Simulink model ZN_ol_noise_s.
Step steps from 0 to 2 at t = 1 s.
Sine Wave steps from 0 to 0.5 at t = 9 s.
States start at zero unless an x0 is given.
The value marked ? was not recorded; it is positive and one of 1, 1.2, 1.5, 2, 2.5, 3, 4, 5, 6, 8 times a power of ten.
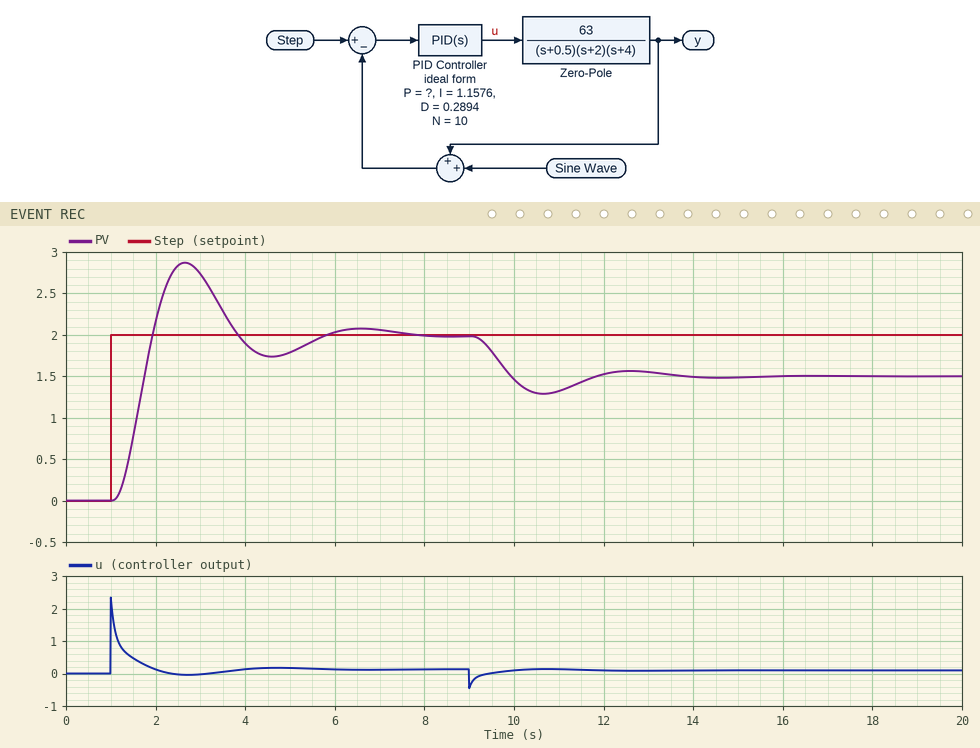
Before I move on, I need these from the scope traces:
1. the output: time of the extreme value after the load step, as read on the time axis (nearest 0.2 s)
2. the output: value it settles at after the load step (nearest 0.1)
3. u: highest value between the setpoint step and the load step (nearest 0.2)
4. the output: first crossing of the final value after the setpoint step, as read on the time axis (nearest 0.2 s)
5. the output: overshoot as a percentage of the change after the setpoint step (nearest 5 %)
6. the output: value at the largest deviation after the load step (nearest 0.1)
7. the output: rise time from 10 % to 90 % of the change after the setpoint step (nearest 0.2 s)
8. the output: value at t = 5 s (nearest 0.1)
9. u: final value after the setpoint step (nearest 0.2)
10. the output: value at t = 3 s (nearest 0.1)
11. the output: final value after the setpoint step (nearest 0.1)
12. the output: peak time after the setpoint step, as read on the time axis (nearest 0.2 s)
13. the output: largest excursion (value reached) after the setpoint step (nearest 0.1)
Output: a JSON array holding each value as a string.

["10.6 s", "1.5", "2.4", "2.0 s", "45 %", "1.3", "0.6 s", "1.8", "0.2", "2.7", "2.0", "2.6 s", "2.9"]
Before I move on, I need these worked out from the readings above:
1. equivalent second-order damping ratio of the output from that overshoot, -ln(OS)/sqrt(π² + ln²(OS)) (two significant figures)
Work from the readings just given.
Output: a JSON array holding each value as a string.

["0.25"]
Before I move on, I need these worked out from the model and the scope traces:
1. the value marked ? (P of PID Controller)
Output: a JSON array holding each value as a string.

["0.3"]
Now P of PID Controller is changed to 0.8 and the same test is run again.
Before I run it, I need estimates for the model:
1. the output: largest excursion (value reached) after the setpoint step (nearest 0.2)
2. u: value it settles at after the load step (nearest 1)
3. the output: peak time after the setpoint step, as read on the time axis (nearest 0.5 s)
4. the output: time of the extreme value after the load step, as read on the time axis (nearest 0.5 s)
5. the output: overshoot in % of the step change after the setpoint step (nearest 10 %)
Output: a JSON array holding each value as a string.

["3.4", "0", "2.0 s", "10.0 s", "70 %"]
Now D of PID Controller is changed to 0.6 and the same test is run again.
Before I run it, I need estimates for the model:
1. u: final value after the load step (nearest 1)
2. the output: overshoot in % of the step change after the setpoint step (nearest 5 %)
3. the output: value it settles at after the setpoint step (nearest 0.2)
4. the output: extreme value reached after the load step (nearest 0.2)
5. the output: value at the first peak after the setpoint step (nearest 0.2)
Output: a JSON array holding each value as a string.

["0", "20 %", "2.0", "1.4", "2.4"]
